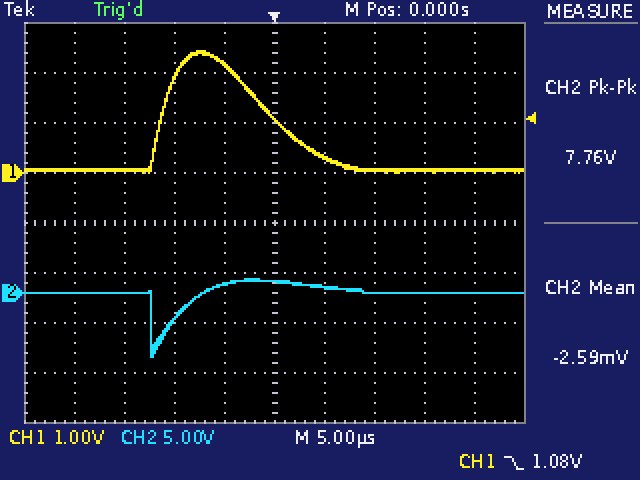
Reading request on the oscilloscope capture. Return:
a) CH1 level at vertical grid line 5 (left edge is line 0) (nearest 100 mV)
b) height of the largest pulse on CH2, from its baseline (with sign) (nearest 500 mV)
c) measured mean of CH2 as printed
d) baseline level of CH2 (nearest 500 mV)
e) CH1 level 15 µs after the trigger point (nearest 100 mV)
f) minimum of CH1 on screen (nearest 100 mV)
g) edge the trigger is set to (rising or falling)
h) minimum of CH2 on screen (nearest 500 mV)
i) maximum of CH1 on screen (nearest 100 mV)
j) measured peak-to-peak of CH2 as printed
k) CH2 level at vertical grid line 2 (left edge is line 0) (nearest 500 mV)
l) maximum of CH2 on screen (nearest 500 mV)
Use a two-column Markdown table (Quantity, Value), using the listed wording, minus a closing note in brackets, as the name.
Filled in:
| Quantity | Value |
|---|---|
| CH1 level at vertical grid line 5 (left edge is line 0) | 1.1 V |
| height of the largest pulse on CH2, from its baseline (with sign) | -6.5 V |
| measured mean of CH2 as printed | -2.59 mV |
| baseline level of CH2 | 0.0 V |
| CH1 level 15 µs after the trigger point | 100 mV |
| minimum of CH1 on screen | 0.0 V |
| edge the trigger is set to | falling |
| minimum of CH2 on screen | -6.5 V |
| maximum of CH1 on screen | 2.4 V |
| measured peak-to-peak of CH2 as printed | 7.76 V |
| CH2 level at vertical grid line 2 (left edge is line 0) | 0.0 V |
| maximum of CH2 on screen | 1.5 V |
